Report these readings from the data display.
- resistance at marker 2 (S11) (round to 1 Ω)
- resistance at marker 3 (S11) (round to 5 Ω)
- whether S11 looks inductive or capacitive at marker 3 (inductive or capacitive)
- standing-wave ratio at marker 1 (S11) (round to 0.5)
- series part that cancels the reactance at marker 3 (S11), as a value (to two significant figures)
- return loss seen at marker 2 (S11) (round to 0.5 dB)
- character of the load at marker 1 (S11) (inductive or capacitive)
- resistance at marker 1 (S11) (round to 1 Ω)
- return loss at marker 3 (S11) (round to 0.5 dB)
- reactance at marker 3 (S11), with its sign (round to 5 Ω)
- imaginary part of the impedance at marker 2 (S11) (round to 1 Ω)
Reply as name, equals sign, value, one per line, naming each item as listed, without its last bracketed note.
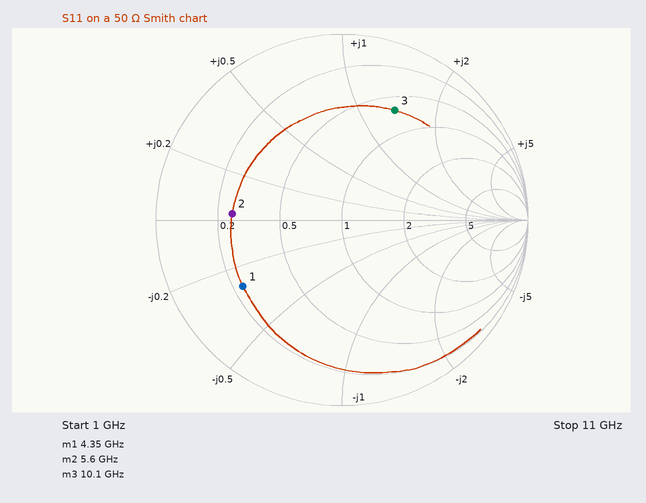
resistance at marker 2 (S11) = 13 Ω
resistance at marker 3 (S11) = 35 Ω
whether S11 looks inductive or capacitive at marker 3 = inductive
standing-wave ratio at marker 1 (S11) = 4.5
series part that cancels the reactance at marker 3 (S11), as a value = 230 fF
return loss seen at marker 2 (S11) = 4.5 dB
character of the load at marker 1 (S11) = capacitive
resistance at marker 1 (S11) = 12 Ω
return loss at marker 3 (S11) = 3.5 dB
reactance at marker 3 (S11), with its sign = +70 Ω
imaginary part of the impedance at marker 2 (S11) = +1 Ω
